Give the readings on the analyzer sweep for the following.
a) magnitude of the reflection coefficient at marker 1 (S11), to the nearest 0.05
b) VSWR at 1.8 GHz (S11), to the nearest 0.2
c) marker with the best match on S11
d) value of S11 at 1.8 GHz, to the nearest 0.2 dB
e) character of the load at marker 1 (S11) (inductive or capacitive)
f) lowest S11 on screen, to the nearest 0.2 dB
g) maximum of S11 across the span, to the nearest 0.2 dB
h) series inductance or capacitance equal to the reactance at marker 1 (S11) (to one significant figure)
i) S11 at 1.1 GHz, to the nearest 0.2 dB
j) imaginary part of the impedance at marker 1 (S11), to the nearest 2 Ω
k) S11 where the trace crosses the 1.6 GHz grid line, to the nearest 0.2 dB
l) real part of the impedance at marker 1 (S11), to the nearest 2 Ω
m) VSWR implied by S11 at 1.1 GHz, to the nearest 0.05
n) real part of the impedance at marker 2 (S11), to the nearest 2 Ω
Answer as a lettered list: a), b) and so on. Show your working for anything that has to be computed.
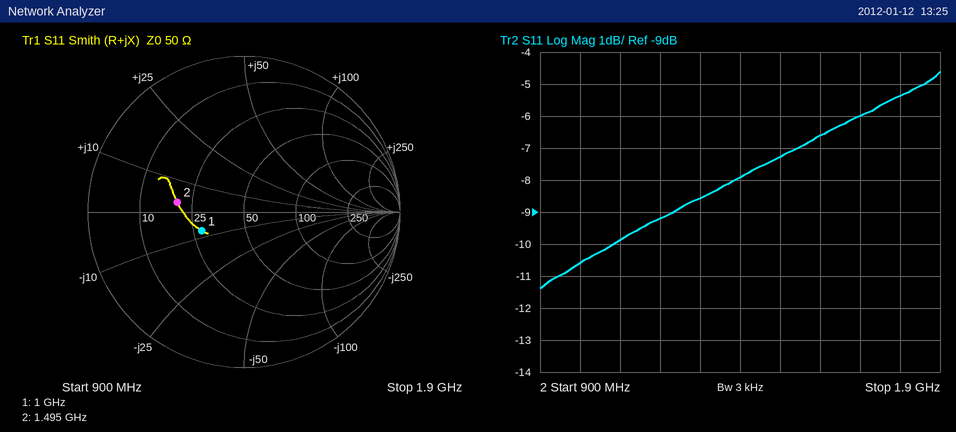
a) 0.30
b) |Γ| = 10^(-5.4/20) = 0.5370; VSWR = (1 + 0.5370)/(1 − 0.5370) ≈ 3.32, so 3.4 to the nearest 0.2
c) marker 1
d) -5.4 dB
e) capacitive
f) -11.4 dB
g) -4.6 dB
h) C = 1/(2π × 1 GHz × 8 Ω) ≈ 20 pF
i) -9.8 dB
j) -8 Ω
k) -6.6 dB
l) 28 Ω
m) |Γ| = 10^(-9.8/20) = 0.3236; VSWR = (1 + 0.3236)/(1 − 0.3236) ≈ 1.96, so 1.95 to the nearest 0.05
n) 20 Ω
